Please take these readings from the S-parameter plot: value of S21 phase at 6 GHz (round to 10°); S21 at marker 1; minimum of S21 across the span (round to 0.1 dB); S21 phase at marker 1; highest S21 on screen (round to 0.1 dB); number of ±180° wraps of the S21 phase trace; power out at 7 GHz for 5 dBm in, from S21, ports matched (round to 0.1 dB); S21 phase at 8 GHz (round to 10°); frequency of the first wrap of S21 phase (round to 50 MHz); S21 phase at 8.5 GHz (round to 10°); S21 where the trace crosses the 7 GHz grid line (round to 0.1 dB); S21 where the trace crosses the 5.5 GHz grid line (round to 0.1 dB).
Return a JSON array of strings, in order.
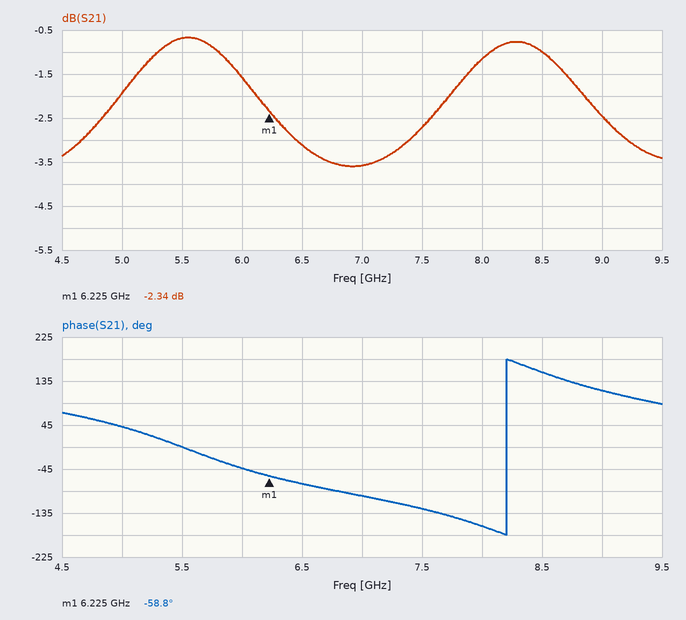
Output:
["-40°", "-2.34 dB", "-3.6 dB", "-58.8°", "-0.7 dB", "1", "1.4 dBm", "-160°", "8.20 GHz", "150°", "-3.6 dB", "-0.7 dB"]
